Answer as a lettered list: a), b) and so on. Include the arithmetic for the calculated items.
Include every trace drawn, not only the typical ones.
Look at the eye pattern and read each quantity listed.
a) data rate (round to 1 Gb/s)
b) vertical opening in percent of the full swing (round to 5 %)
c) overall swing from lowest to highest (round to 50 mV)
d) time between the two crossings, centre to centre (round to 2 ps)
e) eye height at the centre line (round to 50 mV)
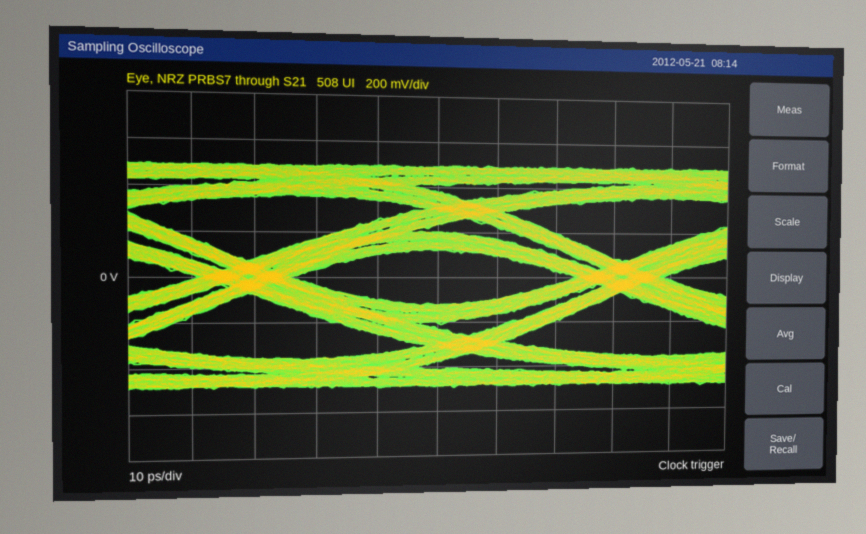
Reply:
a) 16 Gb/s
b) 250 mV / 1.00 V ≈ 25 %
c) 1.00 V
d) 62 ps
e) 250 mV
